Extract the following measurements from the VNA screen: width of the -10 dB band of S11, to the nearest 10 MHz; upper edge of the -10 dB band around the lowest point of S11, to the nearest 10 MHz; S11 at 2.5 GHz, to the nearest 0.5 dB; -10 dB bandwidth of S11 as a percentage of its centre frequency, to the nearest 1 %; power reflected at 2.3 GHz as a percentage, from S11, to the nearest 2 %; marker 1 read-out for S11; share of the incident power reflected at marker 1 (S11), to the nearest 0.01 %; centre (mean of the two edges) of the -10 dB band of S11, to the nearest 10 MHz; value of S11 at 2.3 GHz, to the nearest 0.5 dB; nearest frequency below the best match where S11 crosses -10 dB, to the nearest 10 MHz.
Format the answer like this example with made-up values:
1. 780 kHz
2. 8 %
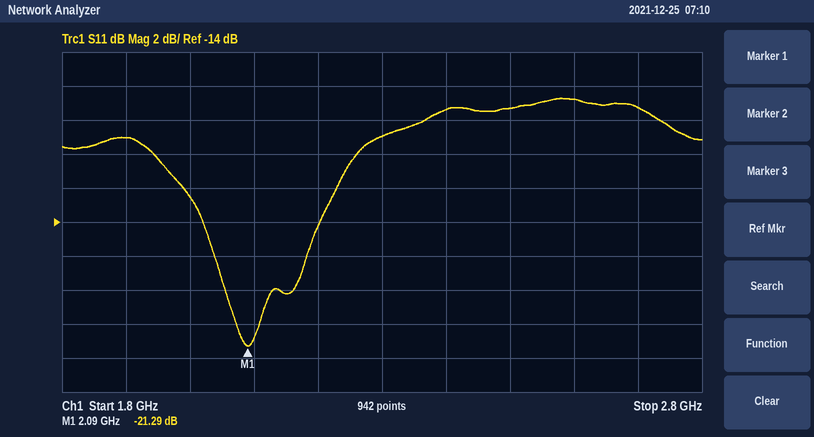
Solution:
1. 320 MHz
2. 2.26 GHz
3. -7.5 dB
4. 15 %
5. 12 %
6. -21.29 dB
7. 0.74 %
8. 2.10 GHz
9. -9.0 dB
10. 1.94 GHz
